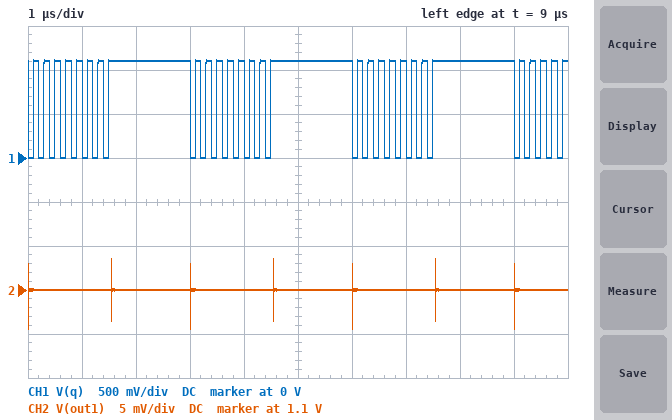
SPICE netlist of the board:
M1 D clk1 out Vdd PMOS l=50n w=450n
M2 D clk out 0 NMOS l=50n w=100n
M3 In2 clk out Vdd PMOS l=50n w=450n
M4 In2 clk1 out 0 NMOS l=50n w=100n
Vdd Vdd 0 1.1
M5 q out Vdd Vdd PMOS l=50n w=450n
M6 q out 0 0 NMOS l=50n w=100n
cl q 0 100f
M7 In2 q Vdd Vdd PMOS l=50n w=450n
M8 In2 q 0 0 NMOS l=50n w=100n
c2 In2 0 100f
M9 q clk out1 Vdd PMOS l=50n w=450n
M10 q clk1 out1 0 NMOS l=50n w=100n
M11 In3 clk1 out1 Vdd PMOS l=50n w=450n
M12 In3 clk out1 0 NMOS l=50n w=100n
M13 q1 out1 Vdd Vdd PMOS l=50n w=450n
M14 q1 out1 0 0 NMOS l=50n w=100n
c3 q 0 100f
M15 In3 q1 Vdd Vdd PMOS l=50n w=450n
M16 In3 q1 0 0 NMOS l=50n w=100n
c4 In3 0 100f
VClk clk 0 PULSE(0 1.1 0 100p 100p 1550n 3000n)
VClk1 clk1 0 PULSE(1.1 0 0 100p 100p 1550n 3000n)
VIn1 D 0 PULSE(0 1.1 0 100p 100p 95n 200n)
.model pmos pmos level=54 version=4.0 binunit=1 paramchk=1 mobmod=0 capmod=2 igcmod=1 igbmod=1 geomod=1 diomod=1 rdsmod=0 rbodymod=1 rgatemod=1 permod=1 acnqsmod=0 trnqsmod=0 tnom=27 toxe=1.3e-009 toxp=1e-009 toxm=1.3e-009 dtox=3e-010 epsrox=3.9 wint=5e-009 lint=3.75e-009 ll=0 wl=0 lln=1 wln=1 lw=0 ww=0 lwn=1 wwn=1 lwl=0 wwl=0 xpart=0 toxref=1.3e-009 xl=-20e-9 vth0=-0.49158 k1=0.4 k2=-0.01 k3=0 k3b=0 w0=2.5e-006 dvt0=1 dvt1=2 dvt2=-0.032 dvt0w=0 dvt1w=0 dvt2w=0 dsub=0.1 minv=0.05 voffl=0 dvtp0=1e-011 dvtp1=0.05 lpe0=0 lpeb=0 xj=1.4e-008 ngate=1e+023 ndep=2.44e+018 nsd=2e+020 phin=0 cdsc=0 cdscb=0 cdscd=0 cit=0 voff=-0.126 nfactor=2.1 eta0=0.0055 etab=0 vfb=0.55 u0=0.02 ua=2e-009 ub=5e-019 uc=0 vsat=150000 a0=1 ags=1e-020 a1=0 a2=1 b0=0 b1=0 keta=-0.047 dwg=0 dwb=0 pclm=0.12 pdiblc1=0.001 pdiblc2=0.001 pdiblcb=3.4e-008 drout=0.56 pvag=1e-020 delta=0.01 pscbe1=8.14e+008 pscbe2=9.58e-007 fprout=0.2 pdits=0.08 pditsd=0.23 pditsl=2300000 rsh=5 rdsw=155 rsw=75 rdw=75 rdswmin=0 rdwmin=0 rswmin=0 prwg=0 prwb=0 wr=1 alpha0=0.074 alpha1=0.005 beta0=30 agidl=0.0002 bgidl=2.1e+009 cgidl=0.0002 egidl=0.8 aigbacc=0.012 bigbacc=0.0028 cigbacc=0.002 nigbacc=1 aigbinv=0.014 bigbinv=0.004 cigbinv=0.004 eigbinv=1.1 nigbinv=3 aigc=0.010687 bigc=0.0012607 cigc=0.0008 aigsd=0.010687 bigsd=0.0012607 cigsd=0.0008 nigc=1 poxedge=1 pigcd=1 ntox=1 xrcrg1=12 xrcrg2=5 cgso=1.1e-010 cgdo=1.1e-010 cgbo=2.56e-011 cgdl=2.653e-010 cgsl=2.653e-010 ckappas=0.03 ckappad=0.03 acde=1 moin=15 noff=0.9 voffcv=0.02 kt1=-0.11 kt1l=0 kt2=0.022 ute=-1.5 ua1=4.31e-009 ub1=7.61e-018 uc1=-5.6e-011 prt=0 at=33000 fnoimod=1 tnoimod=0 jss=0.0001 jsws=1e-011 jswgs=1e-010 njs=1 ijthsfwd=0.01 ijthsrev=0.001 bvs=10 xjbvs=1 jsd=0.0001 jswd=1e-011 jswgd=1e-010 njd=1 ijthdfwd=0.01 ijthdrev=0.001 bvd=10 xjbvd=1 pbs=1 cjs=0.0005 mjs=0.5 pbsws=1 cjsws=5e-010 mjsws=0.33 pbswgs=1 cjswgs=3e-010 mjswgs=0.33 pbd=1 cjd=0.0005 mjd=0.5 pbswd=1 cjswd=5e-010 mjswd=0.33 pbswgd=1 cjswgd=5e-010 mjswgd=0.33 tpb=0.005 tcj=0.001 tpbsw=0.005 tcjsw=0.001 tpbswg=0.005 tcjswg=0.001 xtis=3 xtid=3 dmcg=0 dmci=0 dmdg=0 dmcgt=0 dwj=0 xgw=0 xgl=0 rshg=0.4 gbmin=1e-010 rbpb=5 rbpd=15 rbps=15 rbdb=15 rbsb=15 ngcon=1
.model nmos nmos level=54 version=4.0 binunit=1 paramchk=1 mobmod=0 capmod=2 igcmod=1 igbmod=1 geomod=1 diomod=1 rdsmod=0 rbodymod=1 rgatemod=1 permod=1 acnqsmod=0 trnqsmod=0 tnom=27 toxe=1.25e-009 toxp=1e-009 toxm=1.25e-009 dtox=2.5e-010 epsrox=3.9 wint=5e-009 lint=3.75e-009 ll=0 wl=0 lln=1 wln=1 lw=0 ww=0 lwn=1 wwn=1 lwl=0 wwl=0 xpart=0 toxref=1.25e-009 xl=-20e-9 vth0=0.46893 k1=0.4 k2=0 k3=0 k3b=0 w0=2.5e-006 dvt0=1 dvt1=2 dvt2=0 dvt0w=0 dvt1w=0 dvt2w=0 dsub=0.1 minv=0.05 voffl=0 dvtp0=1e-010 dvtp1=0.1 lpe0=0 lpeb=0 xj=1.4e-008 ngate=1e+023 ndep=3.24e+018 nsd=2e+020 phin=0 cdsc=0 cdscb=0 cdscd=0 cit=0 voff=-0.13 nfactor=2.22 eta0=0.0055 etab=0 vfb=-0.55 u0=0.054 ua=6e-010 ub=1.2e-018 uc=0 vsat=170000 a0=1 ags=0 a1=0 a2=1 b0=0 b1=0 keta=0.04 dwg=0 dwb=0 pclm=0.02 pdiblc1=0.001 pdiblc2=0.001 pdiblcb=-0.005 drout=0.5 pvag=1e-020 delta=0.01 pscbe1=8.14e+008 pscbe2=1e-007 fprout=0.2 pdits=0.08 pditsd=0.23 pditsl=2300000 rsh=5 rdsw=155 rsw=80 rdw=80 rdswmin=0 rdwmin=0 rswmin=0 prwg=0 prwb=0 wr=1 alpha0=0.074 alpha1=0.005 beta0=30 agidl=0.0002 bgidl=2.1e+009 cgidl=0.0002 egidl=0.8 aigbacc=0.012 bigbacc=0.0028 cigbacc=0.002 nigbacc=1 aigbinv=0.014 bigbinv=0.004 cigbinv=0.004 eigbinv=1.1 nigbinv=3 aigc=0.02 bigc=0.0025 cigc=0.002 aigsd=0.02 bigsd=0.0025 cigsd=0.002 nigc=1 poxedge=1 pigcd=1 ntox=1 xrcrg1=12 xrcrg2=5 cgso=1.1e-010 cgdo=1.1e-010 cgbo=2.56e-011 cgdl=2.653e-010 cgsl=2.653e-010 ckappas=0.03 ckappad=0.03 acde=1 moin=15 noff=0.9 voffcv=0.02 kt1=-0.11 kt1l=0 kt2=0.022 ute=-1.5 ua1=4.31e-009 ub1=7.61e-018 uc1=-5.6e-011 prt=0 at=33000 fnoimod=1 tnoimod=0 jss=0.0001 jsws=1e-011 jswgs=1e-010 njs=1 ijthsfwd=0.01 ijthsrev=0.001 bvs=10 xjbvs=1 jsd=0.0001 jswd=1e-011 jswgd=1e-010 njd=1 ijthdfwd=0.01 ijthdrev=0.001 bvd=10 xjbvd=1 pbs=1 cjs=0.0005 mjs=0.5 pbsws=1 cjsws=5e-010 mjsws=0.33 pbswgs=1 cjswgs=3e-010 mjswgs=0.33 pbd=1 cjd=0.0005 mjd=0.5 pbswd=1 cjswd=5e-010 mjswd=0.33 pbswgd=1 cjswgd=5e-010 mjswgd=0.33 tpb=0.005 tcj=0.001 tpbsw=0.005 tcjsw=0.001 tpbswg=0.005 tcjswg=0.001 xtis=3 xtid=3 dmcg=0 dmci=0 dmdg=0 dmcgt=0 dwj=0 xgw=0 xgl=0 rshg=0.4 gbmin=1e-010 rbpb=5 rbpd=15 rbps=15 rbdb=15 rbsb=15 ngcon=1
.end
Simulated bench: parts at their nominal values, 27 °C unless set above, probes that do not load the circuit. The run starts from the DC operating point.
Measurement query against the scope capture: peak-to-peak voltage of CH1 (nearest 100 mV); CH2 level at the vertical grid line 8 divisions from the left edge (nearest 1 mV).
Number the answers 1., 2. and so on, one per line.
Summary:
1. 1.1 V
2. 1.100 V
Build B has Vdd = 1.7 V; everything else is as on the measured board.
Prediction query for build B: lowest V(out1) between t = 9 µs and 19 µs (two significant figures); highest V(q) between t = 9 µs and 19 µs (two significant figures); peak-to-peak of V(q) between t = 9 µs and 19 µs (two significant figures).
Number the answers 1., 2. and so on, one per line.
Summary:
1. 1.6 V
2. 1.7 V
3. 1.2 V
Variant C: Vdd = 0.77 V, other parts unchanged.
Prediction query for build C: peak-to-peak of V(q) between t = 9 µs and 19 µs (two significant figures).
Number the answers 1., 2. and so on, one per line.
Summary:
1. 770 mV
